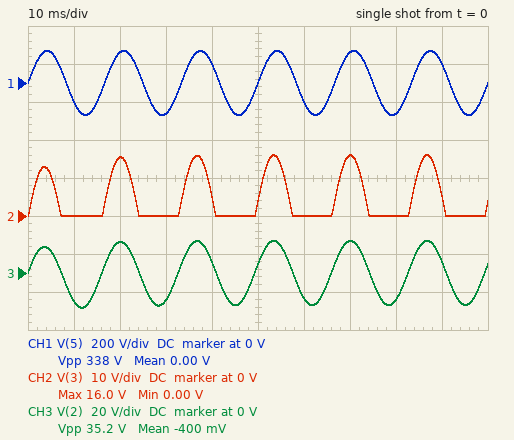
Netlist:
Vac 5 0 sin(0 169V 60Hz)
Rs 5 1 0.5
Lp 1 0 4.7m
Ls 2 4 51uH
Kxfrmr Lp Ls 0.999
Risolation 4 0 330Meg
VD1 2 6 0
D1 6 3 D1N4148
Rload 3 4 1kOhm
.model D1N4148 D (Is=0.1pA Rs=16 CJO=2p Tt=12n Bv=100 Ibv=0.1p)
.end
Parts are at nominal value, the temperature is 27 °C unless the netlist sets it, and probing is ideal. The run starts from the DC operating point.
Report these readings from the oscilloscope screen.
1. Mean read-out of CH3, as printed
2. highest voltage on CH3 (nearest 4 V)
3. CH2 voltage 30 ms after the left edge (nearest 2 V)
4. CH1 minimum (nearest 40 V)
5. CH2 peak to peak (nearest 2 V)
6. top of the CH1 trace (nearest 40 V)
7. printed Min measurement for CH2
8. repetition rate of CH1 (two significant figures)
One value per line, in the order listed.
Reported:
-400 mV
16 V
0 V
-160 V
16 V
160 V
0.00 V
60 Hz
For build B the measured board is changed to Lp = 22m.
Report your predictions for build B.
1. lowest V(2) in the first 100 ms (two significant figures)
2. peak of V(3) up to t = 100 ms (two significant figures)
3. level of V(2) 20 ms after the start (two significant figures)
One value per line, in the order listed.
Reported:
-8.5 V
7.3 V
7.5 V
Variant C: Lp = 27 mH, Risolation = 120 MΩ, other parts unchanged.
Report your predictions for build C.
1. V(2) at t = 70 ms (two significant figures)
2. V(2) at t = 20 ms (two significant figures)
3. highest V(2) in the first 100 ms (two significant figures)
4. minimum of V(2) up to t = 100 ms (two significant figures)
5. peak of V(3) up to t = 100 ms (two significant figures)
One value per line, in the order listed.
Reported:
7.0 V
6.8 V
7.3 V
-7.6 V
6.5 V
